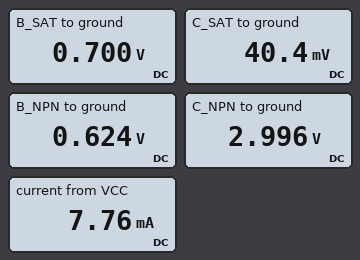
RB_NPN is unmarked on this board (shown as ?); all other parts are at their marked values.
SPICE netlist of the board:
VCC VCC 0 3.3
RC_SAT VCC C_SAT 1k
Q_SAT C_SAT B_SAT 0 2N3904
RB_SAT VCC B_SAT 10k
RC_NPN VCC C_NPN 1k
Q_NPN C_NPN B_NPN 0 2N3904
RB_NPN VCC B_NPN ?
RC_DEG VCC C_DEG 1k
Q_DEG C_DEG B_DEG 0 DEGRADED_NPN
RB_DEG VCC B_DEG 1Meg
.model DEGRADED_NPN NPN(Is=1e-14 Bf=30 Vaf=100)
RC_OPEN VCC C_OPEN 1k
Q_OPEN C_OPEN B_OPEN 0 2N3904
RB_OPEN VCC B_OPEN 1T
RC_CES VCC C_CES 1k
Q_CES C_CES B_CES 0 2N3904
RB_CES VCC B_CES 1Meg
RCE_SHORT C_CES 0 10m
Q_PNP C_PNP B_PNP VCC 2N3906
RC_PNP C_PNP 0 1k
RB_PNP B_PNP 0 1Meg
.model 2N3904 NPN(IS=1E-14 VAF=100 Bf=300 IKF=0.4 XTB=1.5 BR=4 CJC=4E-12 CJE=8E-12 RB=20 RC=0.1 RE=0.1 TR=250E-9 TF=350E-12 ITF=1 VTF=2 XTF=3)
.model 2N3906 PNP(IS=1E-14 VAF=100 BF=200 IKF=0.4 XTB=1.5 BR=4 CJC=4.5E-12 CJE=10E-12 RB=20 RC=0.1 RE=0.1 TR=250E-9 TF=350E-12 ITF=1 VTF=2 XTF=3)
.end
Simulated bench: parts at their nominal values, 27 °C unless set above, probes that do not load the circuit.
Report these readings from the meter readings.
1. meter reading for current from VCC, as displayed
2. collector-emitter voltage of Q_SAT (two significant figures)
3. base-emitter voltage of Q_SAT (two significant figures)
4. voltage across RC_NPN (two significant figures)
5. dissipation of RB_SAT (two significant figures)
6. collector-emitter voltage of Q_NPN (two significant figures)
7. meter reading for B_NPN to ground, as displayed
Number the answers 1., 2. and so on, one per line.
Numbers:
1. 7.76 mA
2. 40 mV
3. 700 mV
4. 300 mV
5. 680 µW
6. 3.0 V
7. 0.624 V
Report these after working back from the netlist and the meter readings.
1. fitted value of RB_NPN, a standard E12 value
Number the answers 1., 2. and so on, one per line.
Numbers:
1. 2.7 MΩ
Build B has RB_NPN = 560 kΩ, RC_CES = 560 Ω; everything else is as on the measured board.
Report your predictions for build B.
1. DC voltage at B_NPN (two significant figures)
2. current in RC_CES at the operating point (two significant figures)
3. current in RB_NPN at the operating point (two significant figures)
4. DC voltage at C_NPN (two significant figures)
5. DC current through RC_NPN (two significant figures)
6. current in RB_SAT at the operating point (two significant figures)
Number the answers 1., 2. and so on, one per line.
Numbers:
1. 660 mV
2. 5.9 mA
3. 4.7 µA
4. 1.9 V
5. 1.4 mA
6. 260 µA
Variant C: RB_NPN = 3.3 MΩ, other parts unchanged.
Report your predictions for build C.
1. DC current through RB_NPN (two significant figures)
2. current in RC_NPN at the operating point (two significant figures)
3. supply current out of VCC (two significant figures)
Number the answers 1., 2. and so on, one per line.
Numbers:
1. 810 nA
2. 250 µA
3. 7.7 mA
